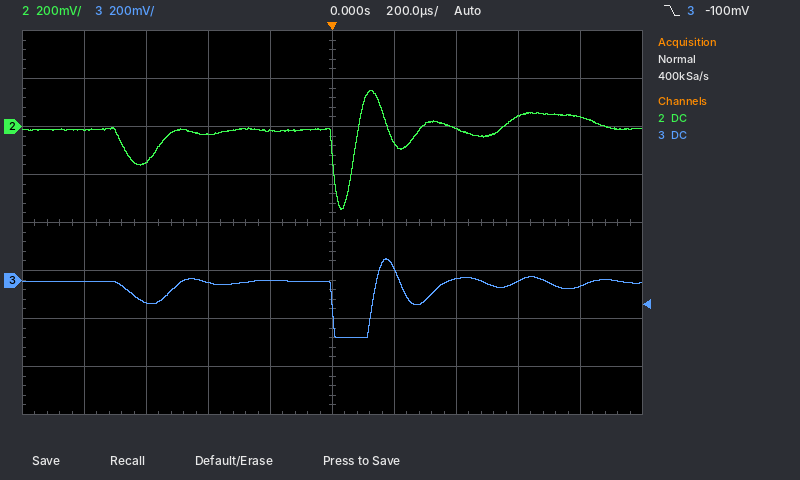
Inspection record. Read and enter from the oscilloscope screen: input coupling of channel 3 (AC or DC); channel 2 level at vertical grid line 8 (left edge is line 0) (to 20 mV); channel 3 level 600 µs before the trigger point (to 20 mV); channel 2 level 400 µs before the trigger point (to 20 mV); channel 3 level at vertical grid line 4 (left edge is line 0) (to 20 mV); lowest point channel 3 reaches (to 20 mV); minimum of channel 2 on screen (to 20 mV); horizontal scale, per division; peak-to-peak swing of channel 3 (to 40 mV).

DC
40 mV
-100 mV
-40 mV
0 mV
-240 mV
-340 mV
200 µs
320 mV
